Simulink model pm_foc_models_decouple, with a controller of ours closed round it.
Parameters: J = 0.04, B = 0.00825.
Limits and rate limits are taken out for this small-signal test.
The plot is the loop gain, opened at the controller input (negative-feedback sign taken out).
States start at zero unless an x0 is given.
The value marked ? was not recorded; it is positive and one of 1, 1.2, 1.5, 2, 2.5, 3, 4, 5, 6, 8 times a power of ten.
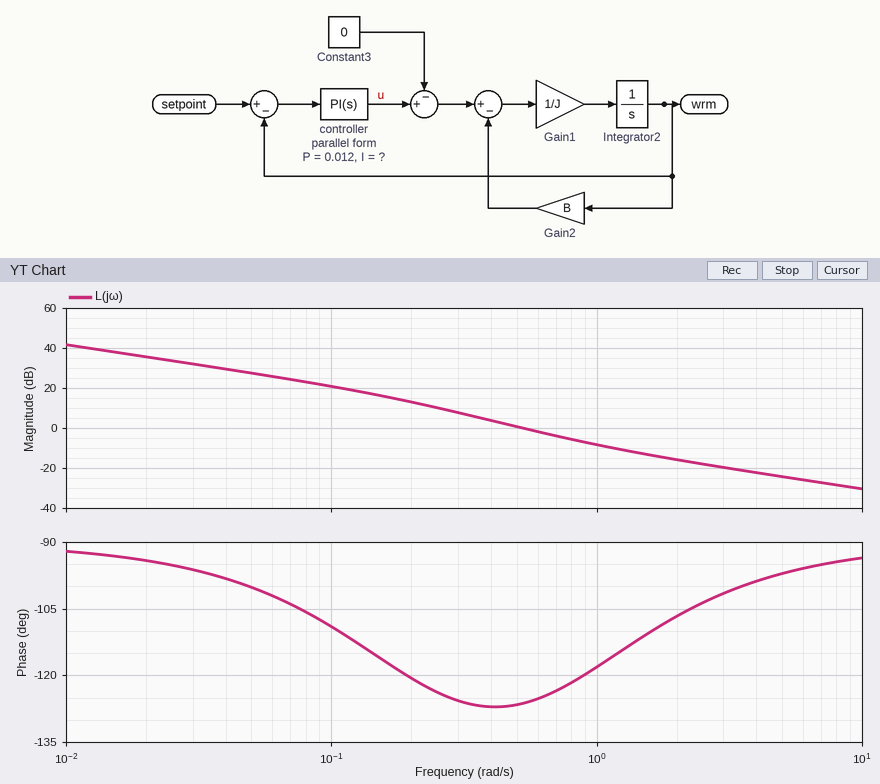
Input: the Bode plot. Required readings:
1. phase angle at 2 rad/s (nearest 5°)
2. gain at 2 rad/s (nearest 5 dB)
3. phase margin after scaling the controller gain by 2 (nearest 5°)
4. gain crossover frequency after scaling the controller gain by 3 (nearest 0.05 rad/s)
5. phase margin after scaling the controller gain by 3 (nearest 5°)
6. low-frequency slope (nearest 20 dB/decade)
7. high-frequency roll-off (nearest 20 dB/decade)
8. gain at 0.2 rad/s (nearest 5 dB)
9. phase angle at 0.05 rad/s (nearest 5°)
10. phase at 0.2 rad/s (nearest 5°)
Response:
-105°
-15 dB
60°
1.10 rad/s
65°
-20 dB/decade
-20 dB/decade
15 dB
-100°
-120°
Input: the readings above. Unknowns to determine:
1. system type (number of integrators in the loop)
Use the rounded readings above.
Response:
1
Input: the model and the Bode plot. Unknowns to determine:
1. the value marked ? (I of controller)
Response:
0.01
